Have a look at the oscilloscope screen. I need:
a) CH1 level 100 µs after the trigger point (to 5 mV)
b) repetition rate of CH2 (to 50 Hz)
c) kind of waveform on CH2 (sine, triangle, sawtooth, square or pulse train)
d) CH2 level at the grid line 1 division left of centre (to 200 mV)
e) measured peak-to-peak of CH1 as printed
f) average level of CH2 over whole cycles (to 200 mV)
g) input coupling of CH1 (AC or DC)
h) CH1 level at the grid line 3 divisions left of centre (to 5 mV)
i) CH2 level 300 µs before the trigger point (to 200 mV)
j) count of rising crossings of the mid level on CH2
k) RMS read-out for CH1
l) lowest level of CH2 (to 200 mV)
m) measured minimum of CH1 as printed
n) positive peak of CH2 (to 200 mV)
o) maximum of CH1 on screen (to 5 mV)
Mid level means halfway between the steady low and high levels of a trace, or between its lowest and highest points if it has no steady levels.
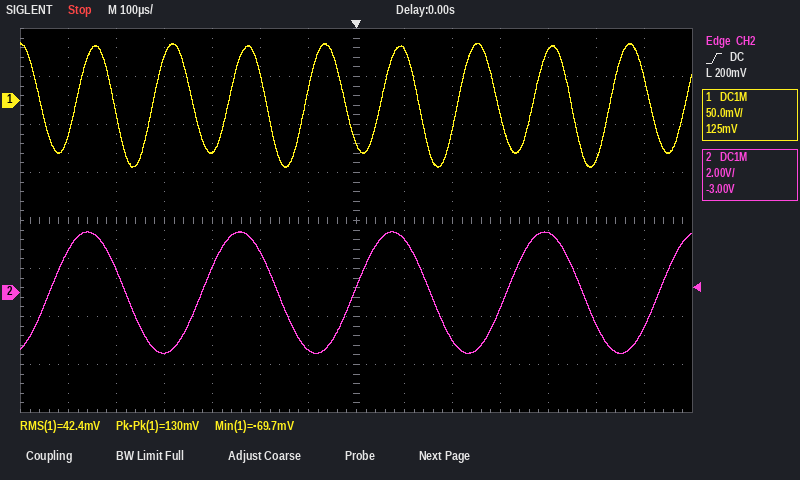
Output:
55 mV
3.15 kHz
sine
-2.4 V
130 mV
0.0 V
DC
-55 mV
1.0 V
5
42.4 mV
-2.6 V
-69.7 mV
2.6 V
60 mV
